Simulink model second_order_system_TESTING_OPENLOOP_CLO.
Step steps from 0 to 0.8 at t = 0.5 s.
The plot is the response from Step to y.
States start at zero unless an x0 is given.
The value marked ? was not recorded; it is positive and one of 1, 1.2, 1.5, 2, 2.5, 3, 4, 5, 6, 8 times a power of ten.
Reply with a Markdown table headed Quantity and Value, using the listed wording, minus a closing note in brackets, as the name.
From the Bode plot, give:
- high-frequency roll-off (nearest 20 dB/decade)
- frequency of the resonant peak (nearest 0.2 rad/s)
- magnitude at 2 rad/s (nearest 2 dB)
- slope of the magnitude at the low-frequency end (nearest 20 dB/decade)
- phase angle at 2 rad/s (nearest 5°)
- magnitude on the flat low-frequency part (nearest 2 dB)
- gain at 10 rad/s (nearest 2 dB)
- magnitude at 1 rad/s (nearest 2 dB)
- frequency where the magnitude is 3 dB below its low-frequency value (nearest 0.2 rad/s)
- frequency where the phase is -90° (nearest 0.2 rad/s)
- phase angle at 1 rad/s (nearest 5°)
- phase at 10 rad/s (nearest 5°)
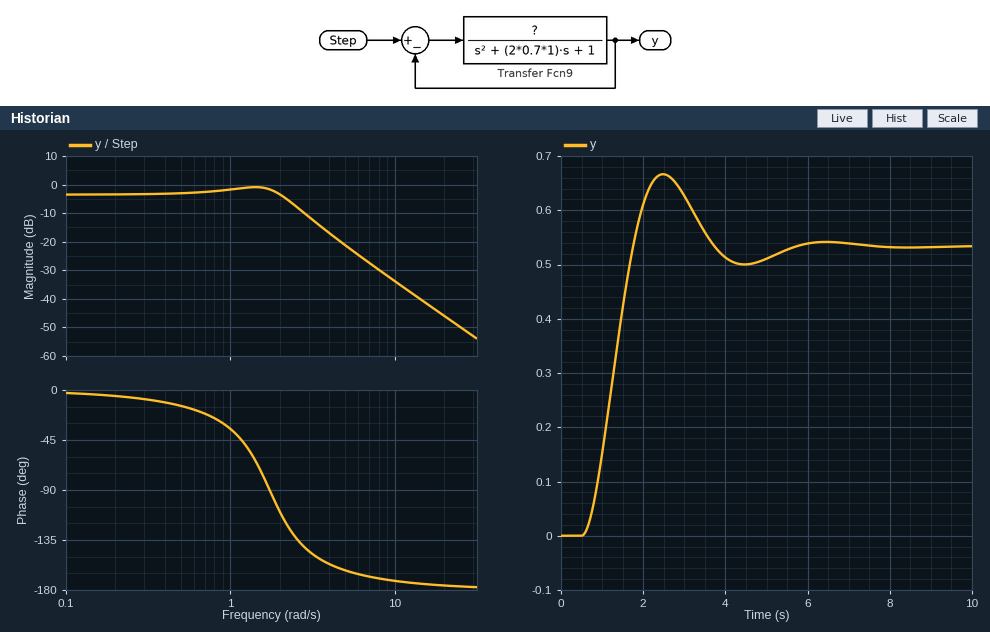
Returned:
| Quantity | Value |
|---|---|
| high-frequency roll-off | -40 dB/decade |
| frequency of the resonant peak | 1.4 rad/s |
| magnitude at 2 rad/s | -4 dB |
| slope of the magnitude at the low-frequency end | 0 dB/decade |
| phase angle at 2 rad/s | -110° |
| magnitude on the flat low-frequency part | -4 dB |
| gain at 10 rad/s | -34 dB |
| magnitude at 1 rad/s | -2 dB |
| frequency where the magnitude is 3 dB below its low-frequency value | 2.4 rad/s |
| frequency where the phase is -90° | 1.8 rad/s |
| phase angle at 1 rad/s | -35° |
| phase at 10 rad/s | -170° |
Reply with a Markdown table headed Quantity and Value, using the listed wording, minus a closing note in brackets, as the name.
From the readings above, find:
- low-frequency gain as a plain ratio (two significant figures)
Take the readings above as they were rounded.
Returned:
| Quantity | Value |
|---|---|
| low-frequency gain as a plain ratio | 0.63 |
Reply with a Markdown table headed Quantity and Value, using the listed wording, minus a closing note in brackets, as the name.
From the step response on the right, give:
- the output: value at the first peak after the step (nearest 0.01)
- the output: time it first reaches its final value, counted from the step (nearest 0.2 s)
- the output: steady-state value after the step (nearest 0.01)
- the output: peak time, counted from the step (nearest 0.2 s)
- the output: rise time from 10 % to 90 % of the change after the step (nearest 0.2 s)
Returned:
| Quantity | Value |
|---|---|
| the output: value at the first peak after the step | 0.67 |
| the output: time it first reaches its final value, counted from the step | 1.2 s |
| the output: steady-state value after the step | 0.53 |
| the output: peak time, counted from the step | 2.0 s |
| the output: rise time from 10 % to 90 % of the change after the step | 0.8 s |
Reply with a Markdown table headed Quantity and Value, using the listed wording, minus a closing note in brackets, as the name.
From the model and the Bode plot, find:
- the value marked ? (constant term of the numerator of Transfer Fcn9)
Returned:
| Quantity | Value |
|---|---|
| the value marked ? | 2 |
